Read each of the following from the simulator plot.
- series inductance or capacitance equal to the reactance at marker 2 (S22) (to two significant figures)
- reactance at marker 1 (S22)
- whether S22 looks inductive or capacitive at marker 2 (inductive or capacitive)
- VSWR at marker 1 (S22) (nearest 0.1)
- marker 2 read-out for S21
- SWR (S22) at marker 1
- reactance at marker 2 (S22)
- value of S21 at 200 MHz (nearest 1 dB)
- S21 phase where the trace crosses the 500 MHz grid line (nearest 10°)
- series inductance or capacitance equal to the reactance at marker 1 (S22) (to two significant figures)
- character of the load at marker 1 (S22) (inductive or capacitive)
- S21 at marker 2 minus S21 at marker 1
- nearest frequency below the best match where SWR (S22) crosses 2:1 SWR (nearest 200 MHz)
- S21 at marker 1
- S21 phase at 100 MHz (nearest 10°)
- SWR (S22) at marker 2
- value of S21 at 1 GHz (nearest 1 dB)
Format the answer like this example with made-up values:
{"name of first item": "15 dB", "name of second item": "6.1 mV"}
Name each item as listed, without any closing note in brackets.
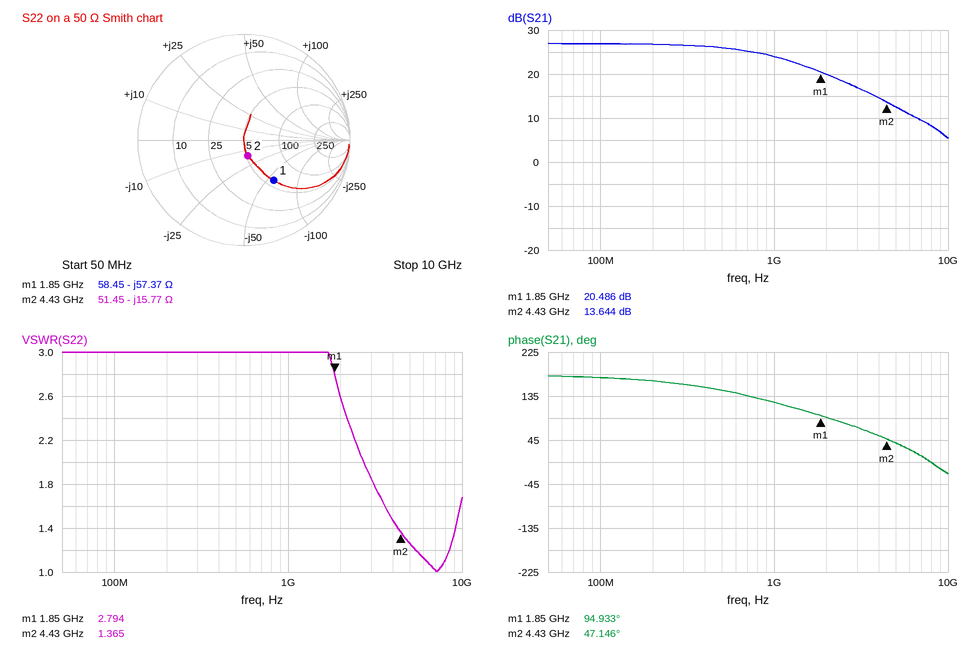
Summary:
{"series inductance or capacitance equal to the reactance at marker 2 (S22)": "2.3 pF", "reactance at marker 1": "-57.37 Ω", "whether S22 looks inductive or capacitive at marker 2": "capacitive", "VSWR at marker 1 (S22)": "2.8", "marker 2 read-out for S21": "13.644 dB", "SWR (S22) at marker 1": "2.794", "reactance at marker 2": "-15.77 Ω", "value of S21 at 200 MHz": "27 dB", "S21 phase where the trace crosses the 500 MHz grid line": "150°", "series inductance or capacitance equal to the reactance at marker 1 (S22)": "1.5 pF", "character of the load at marker 1 (S22)": "capacitive", "S21 at marker 2 minus S21 at marker 1": "-6.842 dB", "nearest frequency below the best match where SWR (S22) crosses 2:1 SWR": "2.8 GHz", "S21 at marker 1": "20.486 dB", "S21 phase at 100 MHz": "170°", "SWR (S22) at marker 2": "1.365", "value of S21 at 1 GHz": "24 dB"}
